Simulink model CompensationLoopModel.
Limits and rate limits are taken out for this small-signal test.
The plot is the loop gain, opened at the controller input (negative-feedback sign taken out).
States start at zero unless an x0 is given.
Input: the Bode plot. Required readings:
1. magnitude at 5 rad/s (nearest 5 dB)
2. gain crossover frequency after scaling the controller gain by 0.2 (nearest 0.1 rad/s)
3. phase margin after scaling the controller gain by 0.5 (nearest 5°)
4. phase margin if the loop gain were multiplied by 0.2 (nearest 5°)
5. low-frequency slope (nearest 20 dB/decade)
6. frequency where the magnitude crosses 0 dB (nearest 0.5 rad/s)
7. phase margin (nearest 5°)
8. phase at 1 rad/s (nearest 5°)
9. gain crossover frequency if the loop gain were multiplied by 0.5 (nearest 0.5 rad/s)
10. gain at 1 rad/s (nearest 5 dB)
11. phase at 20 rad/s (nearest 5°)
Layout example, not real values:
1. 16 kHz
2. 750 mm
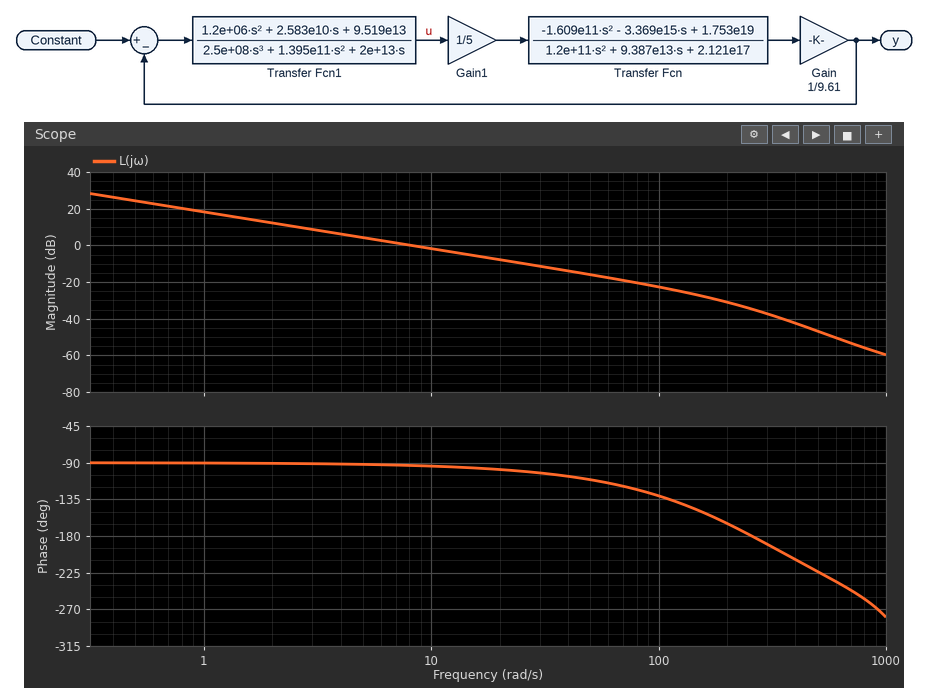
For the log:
1. 5 dB
2. 1.6 rad/s
3. 90°
4. 90°
5. -20 dB/decade
6. 8.0 rad/s
7. 85°
8. -90°
9. 4.0 rad/s
10. 20 dB
11. -100°
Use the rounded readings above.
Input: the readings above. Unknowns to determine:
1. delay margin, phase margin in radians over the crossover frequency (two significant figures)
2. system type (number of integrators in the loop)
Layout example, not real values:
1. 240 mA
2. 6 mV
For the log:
1. 0.19 s
2. 1
